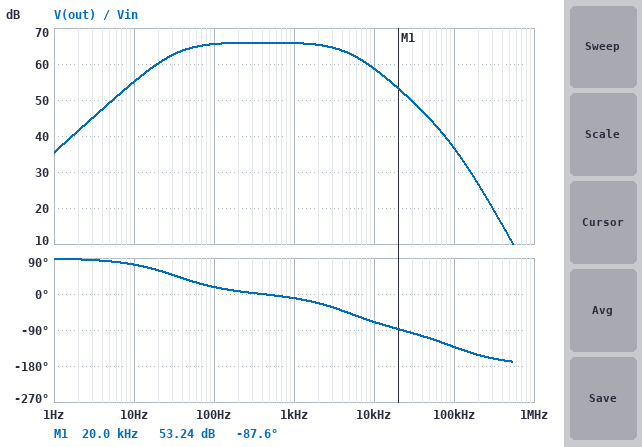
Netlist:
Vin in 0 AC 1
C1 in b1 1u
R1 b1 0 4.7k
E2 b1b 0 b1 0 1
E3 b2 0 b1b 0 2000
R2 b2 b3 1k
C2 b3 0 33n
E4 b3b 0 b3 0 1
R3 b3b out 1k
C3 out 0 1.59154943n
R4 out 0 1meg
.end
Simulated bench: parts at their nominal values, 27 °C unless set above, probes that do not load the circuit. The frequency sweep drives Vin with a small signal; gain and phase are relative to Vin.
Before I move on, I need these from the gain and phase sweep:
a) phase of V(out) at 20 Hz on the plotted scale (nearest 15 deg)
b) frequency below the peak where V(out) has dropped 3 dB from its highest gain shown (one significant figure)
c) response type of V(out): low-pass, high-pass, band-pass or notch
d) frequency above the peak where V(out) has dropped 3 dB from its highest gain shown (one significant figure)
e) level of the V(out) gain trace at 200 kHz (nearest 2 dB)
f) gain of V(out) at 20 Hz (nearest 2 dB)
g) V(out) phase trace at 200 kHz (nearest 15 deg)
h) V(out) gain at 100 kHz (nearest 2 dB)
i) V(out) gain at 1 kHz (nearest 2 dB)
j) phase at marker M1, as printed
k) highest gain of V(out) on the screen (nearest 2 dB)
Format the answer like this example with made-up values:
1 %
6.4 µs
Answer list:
60 deg
30 Hz
band-pass
5 kHz
26 dB
60 dB
-150 deg
36 dB
66 dB
-87.6 deg
66 dB
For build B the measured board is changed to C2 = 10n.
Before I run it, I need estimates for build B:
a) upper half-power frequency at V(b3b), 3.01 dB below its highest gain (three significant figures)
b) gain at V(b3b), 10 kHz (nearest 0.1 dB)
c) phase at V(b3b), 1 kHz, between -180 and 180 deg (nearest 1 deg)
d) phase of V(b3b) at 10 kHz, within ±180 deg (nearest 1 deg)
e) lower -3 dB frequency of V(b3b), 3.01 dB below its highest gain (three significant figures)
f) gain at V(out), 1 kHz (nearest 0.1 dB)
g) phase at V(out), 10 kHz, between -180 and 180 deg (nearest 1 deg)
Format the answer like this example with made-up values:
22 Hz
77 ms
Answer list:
16.0 kHz
64.6 dB
-2 deg
-32 deg
33.7 Hz
66.0 dB
-38 deg
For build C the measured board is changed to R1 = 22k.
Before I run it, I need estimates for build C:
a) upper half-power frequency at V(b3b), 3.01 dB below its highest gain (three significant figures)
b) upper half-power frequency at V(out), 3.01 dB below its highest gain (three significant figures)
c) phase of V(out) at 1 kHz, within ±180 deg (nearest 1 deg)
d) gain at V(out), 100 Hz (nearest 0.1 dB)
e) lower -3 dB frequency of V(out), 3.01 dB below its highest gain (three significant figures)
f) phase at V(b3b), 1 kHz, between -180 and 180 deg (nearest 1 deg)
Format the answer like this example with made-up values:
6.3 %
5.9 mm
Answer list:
4.84 kHz
4.83 kHz
-12 deg
66.0 dB
7.21 Hz
-11 deg
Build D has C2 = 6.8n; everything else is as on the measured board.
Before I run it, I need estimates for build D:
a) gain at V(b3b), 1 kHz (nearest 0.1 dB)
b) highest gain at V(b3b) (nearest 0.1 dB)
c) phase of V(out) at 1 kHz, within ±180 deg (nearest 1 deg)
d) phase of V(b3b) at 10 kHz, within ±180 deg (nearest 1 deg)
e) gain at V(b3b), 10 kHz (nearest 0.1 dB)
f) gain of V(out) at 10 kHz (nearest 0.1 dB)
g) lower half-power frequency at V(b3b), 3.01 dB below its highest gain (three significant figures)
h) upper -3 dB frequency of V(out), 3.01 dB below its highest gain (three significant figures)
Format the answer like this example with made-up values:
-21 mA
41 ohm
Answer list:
66.0 dB
66.0 dB
-1 deg
-23 deg
65.3 dB
65.2 dB
33.8 Hz
22.3 kHz
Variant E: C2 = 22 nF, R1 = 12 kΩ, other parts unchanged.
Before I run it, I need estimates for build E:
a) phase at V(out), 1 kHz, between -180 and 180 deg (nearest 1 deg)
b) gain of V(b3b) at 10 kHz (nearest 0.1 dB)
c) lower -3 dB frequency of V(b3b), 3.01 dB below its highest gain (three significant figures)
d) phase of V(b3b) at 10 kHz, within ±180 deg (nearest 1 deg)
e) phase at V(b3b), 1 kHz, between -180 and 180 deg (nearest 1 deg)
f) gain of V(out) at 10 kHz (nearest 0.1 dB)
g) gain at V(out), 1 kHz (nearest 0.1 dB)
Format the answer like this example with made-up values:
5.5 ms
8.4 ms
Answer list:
-8 deg
61.4 dB
13.2 Hz
-54 deg
-7 deg
61.3 dB
65.9 dB
